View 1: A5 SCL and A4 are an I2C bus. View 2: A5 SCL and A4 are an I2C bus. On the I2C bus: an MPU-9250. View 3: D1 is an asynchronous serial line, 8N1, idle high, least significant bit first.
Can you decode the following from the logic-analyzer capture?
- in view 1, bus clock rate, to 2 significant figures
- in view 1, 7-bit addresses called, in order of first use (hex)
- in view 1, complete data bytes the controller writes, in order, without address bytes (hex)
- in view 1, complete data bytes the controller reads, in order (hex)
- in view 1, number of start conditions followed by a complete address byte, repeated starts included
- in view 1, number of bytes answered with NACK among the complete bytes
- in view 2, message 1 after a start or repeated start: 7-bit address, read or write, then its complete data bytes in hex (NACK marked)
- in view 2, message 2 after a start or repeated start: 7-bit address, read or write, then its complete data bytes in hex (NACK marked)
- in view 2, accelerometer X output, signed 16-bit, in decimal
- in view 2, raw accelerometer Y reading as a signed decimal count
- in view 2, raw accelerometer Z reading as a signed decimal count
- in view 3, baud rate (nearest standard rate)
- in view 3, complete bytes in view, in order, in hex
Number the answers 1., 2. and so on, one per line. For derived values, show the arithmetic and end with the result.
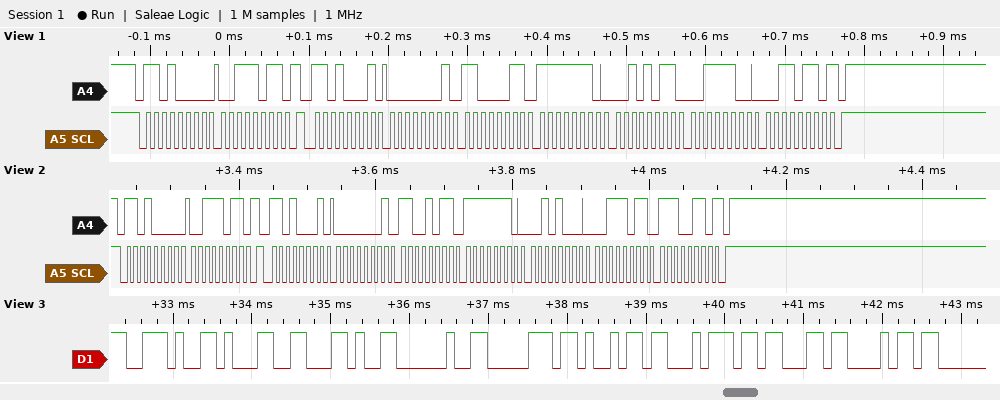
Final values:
1. 100 kHz
2. 0x68
3. 3B
4. 01 C3 FE 2B 3C 36
5. 2
6. 1
7. 0x68 write: 3B
8. 0x68 read: 01 CB FE 28 3B E6 NACK
9. 0x01CB = 459
10. 0xFE28 = -472
11. 0x3BE6 = 15334
12. 9600 baud
13. 0x2E 0x31 0x2C 0x20 0x70 0x69 0x74 0x63 0x68
